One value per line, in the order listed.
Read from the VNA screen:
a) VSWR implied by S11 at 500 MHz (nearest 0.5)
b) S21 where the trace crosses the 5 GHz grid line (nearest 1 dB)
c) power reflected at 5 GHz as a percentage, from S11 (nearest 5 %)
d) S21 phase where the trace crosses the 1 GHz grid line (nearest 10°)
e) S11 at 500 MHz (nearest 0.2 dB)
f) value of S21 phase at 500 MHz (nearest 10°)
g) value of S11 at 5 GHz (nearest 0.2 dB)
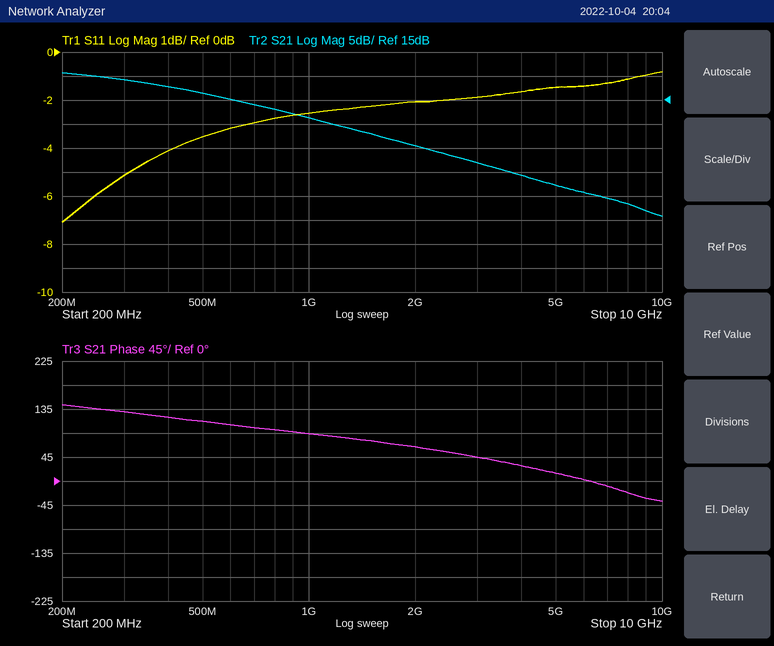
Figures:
5.0
-3 dB
70 %
90°
-3.6 dB
110°
-1.4 dB
